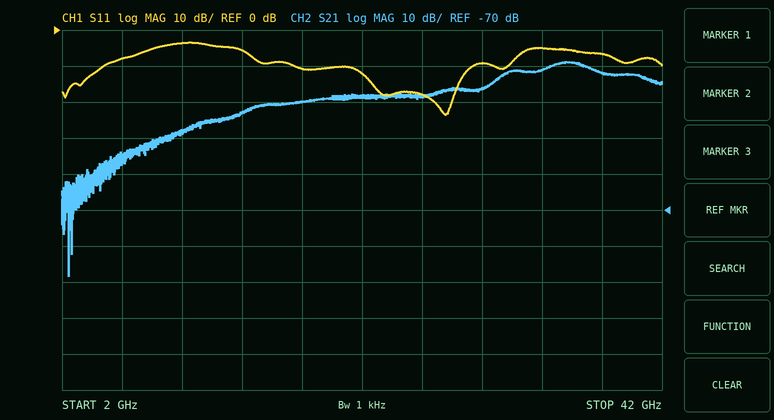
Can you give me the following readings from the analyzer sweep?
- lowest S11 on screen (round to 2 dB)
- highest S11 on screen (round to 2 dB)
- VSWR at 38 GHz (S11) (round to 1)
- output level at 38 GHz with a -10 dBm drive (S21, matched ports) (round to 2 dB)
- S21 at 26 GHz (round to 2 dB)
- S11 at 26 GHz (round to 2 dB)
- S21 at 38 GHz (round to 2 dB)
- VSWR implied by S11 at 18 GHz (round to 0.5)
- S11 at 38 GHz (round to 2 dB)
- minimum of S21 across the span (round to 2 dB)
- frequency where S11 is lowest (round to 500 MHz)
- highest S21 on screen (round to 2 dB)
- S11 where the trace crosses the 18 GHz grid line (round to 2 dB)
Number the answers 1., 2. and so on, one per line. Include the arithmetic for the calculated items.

1. -24 dB
2. -4 dB
3. |Γ| = 10^(-6/20) = 0.5012; VSWR = (1 + 0.5012)/(1 − 0.5012) ≈ 3
4. -10 dBm + (-32 dB) = -42 dBm
5. -38 dB
6. -18 dB
7. -32 dB
8. |Γ| = 10^(-10/20) = 0.3162; VSWR = (1 + 0.3162)/(1 − 0.3162) ≈ 1.92, so 2.0 to the nearest 0.5
9. -6 dB
10. -88 dB
11. 27.5 GHz
12. -28 dB
13. -10 dB
